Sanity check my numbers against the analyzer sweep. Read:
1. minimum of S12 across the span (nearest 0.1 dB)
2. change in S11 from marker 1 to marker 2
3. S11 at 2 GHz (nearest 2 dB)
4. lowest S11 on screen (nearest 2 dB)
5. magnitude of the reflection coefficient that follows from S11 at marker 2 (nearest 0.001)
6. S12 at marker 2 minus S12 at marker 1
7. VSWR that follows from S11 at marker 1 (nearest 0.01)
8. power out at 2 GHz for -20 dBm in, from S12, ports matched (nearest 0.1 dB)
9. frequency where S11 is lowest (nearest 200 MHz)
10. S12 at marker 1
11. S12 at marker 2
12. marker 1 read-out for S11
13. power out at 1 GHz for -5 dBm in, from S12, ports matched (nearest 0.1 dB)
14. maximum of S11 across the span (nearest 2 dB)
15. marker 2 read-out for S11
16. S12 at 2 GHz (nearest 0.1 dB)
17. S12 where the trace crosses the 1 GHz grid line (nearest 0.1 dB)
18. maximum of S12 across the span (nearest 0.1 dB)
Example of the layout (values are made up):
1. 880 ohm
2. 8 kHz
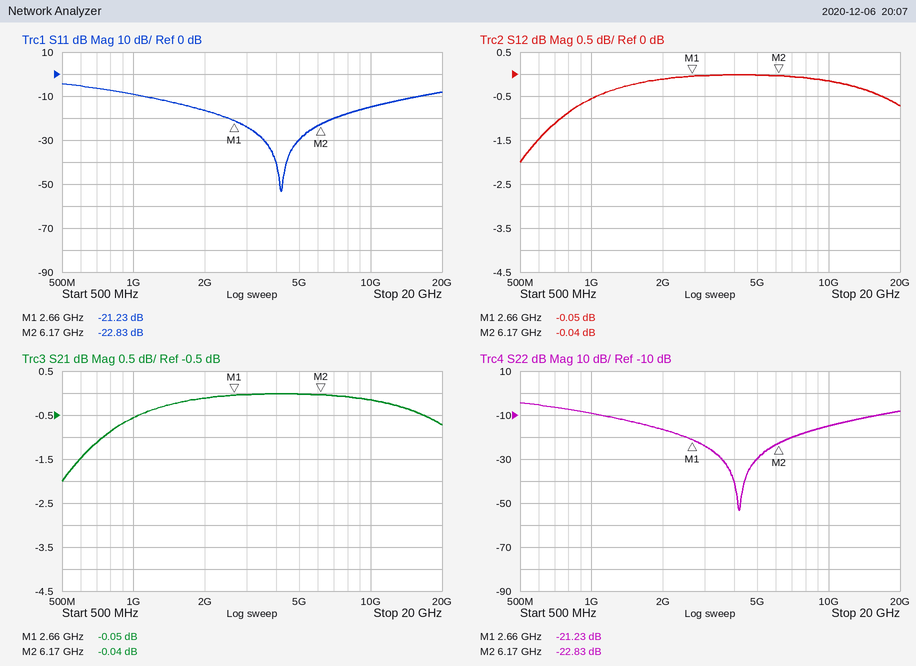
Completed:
1. -2.0 dB
2. -1.60 dB
3. -16 dB
4. -54 dB
5. 0.072
6. 0.01 dB
7. 1.19
8. -20.1 dBm
9. 4.2 GHz
10. -0.05 dB
11. -0.04 dB
12. -21.23 dB
13. -5.6 dBm
14. -4 dB
15. -22.83 dB
16. -0.1 dB
17. -0.6 dB
18. 0.0 dB
